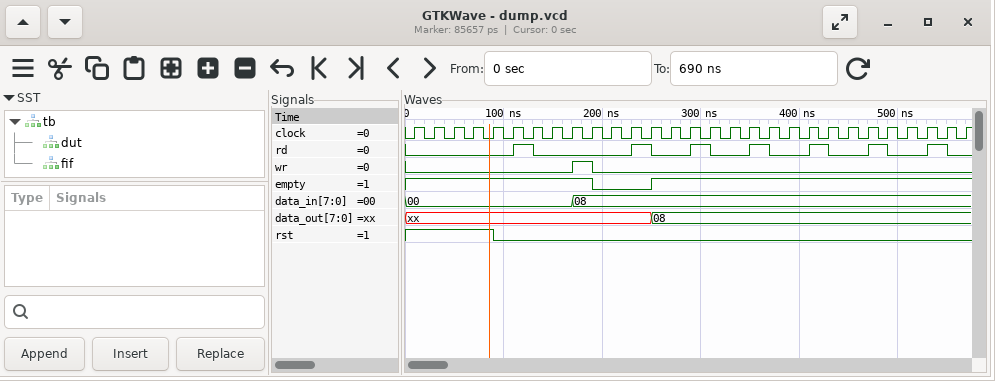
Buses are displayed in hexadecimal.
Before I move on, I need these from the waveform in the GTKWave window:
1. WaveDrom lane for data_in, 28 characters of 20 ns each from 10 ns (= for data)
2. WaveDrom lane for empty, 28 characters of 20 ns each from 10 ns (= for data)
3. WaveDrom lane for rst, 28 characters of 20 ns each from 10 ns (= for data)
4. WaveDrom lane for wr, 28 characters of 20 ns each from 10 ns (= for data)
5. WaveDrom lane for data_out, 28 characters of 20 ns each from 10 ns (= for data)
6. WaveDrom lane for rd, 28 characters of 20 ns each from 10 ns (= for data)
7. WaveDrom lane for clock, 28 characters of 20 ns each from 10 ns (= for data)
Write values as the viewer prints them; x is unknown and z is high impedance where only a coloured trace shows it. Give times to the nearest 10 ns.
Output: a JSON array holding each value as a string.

["{name: 'data_in', wave: '=.......=...................', data: '00 08'}", "{name: 'empty', wave: '1........0..1...............'}", "{name: 'rst', wave: '1...0.......................'}", "{name: 'wr', wave: '0.......10..................'}", "{name: 'data_out', wave: 'x...........=...............', data: '08'}", "{name: 'rd', wave: '0....10....10.10.10.10.10.10'}", "{name: 'clock', wave: 'p...........................'}"]
